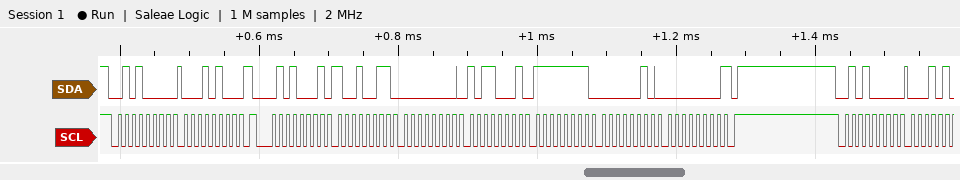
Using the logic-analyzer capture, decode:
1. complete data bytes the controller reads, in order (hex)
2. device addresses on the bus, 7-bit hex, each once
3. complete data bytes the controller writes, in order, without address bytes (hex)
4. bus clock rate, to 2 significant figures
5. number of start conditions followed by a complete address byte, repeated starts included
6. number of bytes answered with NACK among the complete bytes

93 00 B1 FF 02 00
0x28
14
100 kHz
3
1
